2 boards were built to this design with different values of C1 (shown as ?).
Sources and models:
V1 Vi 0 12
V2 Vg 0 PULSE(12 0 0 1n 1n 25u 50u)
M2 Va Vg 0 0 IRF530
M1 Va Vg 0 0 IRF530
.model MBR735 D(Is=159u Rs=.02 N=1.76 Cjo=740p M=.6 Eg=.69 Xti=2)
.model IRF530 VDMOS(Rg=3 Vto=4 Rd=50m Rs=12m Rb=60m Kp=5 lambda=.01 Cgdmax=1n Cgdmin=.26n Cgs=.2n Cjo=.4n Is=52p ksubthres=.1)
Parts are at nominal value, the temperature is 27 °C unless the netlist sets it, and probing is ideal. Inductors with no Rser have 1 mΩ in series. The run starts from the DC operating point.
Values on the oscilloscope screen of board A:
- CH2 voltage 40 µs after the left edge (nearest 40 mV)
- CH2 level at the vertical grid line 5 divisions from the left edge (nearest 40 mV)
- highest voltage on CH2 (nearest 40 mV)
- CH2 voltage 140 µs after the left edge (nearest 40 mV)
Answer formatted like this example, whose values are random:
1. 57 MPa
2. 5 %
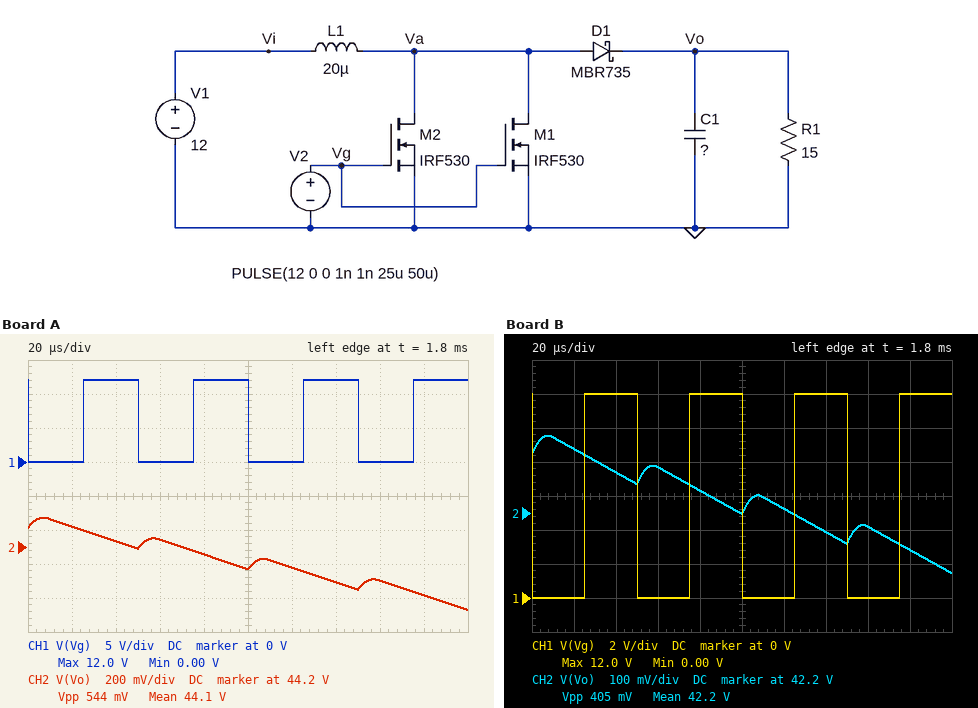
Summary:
1. 44.24 V
2. 44.08 V
3. 44.36 V
4. 44.00 V
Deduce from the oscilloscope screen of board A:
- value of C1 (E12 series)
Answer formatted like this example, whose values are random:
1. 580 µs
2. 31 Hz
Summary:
1. 680 µF
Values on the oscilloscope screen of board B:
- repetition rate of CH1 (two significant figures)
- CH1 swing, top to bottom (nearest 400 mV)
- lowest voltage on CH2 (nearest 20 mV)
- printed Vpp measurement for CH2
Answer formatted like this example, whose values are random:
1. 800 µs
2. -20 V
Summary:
1. 20 kHz
2. 12.0 V
3. 42.02 V
4. 405 mV
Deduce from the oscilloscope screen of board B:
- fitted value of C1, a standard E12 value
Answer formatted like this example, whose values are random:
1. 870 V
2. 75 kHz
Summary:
1. 820 µF
